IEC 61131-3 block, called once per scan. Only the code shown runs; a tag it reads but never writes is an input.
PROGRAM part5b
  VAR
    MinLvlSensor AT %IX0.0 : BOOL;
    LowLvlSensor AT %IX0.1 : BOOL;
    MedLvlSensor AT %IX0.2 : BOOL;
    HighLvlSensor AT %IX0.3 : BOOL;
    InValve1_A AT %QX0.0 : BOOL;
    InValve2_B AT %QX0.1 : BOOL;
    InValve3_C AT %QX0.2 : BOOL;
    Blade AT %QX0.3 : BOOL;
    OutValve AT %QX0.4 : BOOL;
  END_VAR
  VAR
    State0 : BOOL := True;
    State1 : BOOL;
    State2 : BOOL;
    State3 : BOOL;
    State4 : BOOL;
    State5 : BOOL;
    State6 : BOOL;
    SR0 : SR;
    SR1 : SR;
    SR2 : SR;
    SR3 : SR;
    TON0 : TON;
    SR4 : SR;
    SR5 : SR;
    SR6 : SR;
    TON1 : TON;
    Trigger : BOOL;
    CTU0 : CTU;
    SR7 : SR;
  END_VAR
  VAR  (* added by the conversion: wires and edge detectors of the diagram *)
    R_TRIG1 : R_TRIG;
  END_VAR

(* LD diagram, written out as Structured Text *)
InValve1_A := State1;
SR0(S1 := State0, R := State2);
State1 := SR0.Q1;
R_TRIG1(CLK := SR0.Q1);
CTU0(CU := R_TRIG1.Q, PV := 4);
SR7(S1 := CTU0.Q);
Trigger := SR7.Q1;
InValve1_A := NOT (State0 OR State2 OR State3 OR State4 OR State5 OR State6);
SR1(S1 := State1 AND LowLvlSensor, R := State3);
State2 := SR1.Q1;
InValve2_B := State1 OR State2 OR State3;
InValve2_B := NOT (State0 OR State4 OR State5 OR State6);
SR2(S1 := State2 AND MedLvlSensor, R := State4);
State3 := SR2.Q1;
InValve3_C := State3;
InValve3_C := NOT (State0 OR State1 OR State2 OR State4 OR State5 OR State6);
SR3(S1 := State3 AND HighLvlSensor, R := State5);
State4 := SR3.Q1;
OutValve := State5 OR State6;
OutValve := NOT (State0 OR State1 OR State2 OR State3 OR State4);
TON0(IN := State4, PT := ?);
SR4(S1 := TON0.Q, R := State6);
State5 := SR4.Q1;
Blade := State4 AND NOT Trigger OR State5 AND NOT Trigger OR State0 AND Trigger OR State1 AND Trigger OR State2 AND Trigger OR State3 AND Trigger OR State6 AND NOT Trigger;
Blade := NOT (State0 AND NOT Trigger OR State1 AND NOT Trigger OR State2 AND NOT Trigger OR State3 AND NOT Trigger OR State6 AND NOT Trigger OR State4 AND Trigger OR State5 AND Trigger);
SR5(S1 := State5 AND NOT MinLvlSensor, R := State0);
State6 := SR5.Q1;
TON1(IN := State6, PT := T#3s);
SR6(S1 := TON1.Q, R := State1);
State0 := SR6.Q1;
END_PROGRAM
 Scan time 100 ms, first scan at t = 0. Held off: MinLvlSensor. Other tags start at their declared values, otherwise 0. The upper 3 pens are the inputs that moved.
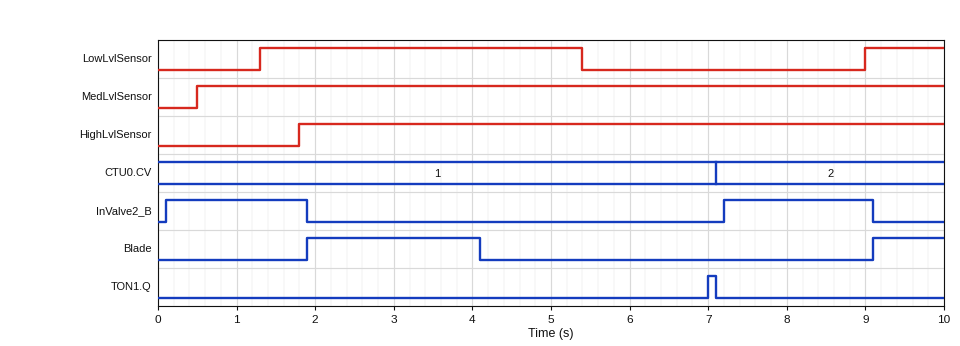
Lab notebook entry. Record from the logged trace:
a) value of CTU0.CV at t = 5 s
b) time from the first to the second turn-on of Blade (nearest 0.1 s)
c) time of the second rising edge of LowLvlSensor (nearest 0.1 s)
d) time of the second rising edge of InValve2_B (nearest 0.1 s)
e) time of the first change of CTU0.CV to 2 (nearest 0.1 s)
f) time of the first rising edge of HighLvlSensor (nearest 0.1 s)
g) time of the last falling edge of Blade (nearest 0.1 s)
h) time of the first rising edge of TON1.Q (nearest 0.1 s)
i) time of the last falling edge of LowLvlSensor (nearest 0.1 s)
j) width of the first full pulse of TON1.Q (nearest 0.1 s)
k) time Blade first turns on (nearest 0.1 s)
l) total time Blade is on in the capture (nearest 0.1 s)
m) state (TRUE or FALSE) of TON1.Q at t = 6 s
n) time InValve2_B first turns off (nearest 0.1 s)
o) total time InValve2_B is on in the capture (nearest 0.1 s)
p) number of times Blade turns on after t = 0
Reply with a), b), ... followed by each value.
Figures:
a) 1
b) 7.2 s
c) 9.0 s
d) 7.2 s
e) 7.1 s
f) 1.8 s
g) 4.1 s
h) 7.0 s
i) 5.4 s
j) 0.1 s
k) 1.9 s
l) 3.1 s
m) FALSE
n) 1.9 s
o) 3.7 s
p) 2
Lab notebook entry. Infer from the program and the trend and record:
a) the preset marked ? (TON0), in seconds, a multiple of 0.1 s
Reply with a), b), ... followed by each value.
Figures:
a) 2.2 s
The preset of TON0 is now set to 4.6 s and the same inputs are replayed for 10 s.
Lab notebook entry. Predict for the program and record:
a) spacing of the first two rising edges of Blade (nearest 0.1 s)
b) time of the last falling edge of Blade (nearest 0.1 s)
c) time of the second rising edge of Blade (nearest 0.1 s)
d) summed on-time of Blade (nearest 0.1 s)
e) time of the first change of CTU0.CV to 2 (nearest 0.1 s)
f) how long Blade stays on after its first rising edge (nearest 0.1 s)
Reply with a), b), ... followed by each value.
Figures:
a) 7.7 s
b) 6.5 s
c) 9.6 s
d) 5.0 s
e) 9.5 s
f) 4.6 s
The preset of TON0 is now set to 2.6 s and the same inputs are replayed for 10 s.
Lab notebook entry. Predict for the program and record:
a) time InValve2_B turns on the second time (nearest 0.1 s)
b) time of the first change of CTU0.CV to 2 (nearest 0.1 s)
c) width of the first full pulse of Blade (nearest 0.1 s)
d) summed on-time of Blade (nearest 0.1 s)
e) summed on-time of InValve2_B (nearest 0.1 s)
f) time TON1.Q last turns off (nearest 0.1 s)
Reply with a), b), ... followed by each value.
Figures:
a) 7.6 s
b) 7.5 s
c) 2.6 s
d) 3.5 s
e) 3.3 s
f) 7.5 s
